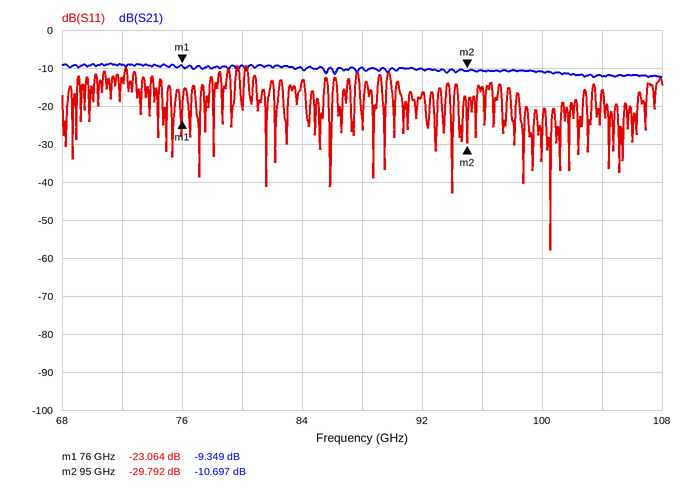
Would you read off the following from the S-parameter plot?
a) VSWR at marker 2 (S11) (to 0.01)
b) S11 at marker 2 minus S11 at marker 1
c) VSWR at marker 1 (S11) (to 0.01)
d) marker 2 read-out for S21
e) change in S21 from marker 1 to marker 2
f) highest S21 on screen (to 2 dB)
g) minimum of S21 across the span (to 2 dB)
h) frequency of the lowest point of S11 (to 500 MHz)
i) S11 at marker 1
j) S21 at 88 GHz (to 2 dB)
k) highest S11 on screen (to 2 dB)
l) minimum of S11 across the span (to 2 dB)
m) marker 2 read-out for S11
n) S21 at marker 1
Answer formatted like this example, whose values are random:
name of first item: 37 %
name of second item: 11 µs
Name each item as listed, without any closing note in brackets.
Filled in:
VSWR at marker 2 (S11): 1.07
S11 at marker 2 minus S11 at marker 1: -6.728 dB
VSWR at marker 1 (S11): 1.15
marker 2 read-out for S21: -10.697 dB
change in S21 from marker 1 to marker 2: -1.348 dB
highest S21 on screen: -8 dB
minimum of S21 across the span: -12 dB
frequency of the lowest point of S11: 100.5 GHz
S11 at marker 1: -23.064 dB
S21 at 88 GHz: -10 dB
highest S11 on screen: -10 dB
minimum of S11 across the span: -58 dB
marker 2 read-out for S11: -29.792 dB
S21 at marker 1: -9.349 dB
